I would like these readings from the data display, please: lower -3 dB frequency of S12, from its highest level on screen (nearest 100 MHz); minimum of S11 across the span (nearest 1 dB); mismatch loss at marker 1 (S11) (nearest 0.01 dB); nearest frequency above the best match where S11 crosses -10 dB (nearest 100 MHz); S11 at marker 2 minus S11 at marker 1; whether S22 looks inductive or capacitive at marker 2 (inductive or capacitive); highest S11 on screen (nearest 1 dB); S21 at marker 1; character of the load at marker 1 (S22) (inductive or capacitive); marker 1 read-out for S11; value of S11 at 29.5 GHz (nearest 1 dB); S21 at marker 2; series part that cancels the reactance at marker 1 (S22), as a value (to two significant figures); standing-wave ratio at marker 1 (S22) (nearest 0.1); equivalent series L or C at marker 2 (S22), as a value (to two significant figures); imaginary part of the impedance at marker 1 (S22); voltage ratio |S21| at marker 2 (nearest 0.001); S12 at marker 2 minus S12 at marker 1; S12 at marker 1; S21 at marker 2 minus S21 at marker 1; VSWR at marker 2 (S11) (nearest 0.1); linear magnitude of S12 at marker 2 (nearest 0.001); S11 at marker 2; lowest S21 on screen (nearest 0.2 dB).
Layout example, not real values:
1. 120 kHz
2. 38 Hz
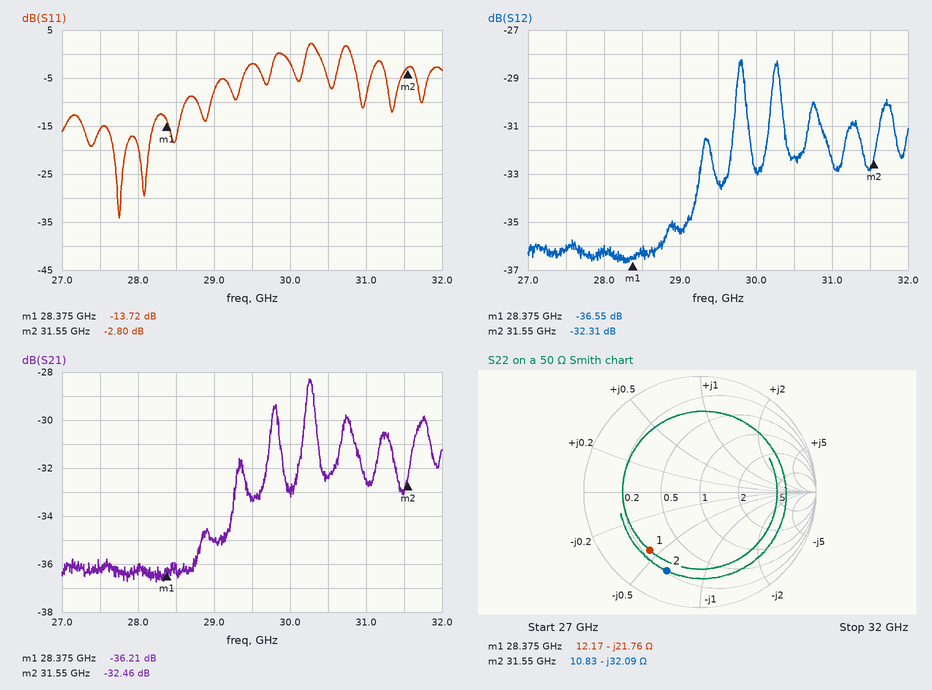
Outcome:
1. 29.7 GHz
2. -34 dB
3. 0.19 dB
4. 28.6 GHz
5. 10.92 dB
6. capacitive
7. 2 dB
8. -36.21 dB
9. capacitive
10. -13.72 dB
11. -2 dB
12. -32.46 dB
13. 120 pH
14. 4.9
15. 160 fF
16. -21.76 Ω
17. 0.024
18. 4.24 dB
19. -36.55 dB
20. 3.75 dB
21. 6.3
22. 0.024
23. -2.80 dB
24. -36.8 dB
